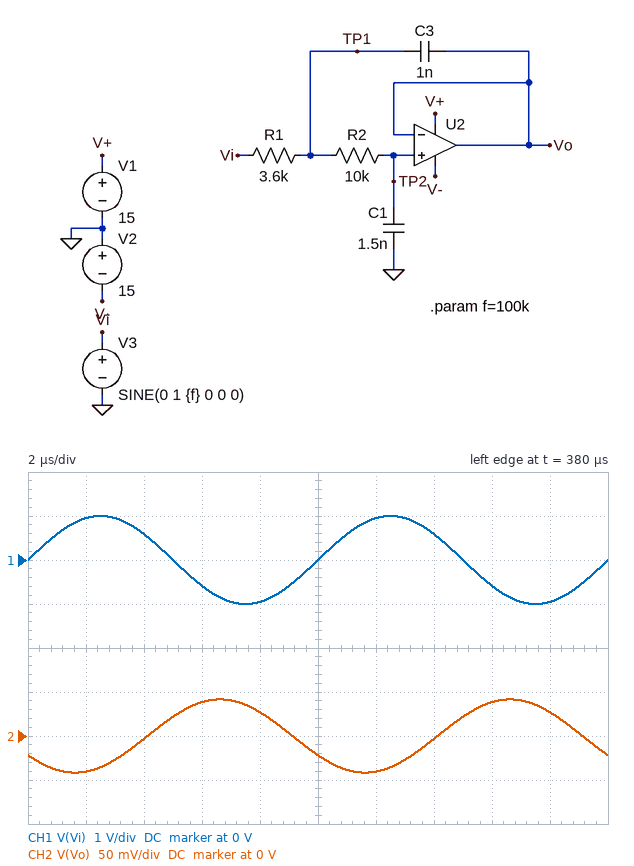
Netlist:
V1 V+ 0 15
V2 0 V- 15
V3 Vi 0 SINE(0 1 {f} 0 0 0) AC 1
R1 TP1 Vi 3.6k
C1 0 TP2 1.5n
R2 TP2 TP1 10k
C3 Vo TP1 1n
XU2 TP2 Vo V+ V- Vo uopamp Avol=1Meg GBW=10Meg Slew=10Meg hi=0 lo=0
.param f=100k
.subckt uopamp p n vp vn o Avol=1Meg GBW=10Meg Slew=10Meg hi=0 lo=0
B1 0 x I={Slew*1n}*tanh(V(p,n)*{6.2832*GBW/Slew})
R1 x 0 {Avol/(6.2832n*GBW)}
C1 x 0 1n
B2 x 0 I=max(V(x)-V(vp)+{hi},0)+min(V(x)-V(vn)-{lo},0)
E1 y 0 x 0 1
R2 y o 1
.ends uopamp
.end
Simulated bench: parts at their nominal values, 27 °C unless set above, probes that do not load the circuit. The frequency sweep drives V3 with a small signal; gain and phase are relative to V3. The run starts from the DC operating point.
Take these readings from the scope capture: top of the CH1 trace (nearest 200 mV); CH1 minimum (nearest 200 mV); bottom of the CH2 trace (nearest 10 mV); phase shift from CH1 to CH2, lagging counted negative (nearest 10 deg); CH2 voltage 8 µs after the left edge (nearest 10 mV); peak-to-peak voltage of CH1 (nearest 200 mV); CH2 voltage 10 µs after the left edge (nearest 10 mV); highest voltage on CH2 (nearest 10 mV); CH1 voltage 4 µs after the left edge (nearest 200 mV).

1.0 V
-1.0 V
-40 mV
-150 deg
30 mV
2.0 V
-20 mV
40 mV
600 mV
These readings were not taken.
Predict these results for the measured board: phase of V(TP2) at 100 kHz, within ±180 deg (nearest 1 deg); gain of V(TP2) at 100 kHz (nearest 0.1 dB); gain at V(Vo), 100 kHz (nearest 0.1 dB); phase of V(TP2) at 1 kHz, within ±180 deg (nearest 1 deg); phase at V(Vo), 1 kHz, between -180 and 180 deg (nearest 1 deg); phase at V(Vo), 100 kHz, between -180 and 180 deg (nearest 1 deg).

-148 deg
-27.6 dB
-27.6 dB
-7 deg
-7 deg
-148 deg
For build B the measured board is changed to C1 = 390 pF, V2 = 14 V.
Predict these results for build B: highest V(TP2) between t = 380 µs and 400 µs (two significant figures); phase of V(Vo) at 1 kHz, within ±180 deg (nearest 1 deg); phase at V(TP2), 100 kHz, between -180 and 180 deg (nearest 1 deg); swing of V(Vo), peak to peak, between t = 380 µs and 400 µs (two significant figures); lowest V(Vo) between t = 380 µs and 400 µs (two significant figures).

180 mV
-2 deg
-144 deg
350 mV
-180 mV
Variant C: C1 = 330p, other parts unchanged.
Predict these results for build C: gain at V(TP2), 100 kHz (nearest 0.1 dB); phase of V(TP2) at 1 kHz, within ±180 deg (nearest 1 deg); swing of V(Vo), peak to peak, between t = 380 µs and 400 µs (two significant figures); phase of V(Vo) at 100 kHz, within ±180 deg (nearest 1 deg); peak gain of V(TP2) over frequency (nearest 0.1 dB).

-13.4 dB
-2 deg
430 mV
-143 deg
0.1 dB
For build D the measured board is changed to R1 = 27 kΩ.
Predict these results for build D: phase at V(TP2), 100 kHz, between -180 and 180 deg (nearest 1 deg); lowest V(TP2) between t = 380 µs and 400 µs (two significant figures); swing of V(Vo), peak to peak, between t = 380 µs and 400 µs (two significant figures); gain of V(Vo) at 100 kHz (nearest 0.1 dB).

-168 deg
-6.1 mV
12 mV
-44.2 dB
